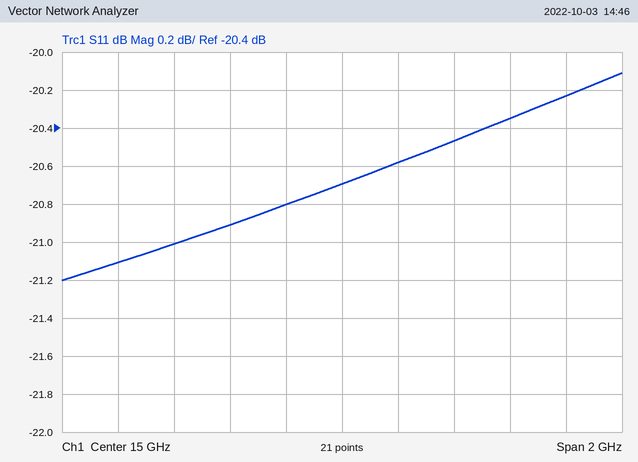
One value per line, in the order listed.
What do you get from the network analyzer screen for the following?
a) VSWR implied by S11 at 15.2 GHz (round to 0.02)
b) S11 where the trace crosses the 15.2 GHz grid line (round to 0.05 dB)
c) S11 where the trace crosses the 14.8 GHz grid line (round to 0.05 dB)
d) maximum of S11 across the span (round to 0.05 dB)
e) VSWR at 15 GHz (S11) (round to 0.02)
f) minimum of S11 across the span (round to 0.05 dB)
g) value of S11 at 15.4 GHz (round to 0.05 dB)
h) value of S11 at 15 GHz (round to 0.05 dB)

1.20
-20.60 dB
-20.80 dB
-20.10 dB
1.20
-21.20 dB
-20.45 dB
-20.70 dB
